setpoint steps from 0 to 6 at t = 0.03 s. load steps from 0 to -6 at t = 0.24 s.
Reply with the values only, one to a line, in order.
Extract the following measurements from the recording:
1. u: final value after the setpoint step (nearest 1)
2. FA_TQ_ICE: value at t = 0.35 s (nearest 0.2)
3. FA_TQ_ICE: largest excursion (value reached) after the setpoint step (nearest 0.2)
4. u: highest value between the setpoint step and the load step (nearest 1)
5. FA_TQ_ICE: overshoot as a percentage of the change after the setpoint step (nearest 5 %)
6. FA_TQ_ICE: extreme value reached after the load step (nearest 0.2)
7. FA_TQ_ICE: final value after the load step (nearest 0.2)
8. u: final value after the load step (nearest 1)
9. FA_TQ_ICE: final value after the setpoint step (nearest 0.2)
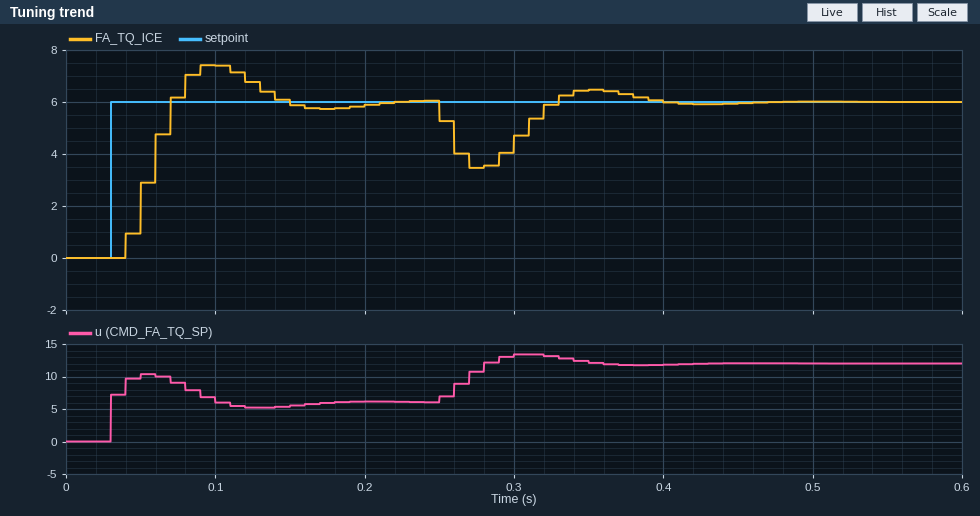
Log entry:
6
6.4
7.4
10
25 %
3.4
6.0
12
6.0
